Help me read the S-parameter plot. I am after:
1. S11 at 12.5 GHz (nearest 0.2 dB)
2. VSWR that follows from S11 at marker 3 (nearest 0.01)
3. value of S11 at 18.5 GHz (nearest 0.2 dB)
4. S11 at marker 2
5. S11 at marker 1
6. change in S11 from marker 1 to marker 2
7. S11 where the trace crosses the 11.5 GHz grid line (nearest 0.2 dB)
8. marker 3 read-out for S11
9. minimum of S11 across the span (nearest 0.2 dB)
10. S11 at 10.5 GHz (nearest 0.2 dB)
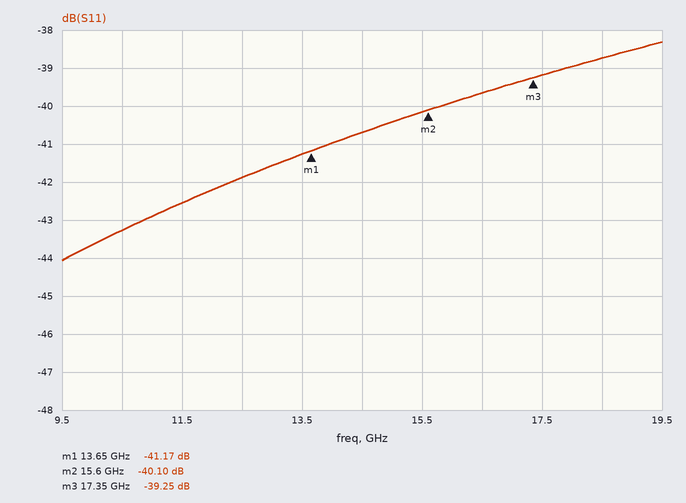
-41.8 dB
1.02
-38.8 dB
-40.10 dB
-41.17 dB
1.07 dB
-42.6 dB
-39.25 dB
-44.0 dB
-43.2 dB
